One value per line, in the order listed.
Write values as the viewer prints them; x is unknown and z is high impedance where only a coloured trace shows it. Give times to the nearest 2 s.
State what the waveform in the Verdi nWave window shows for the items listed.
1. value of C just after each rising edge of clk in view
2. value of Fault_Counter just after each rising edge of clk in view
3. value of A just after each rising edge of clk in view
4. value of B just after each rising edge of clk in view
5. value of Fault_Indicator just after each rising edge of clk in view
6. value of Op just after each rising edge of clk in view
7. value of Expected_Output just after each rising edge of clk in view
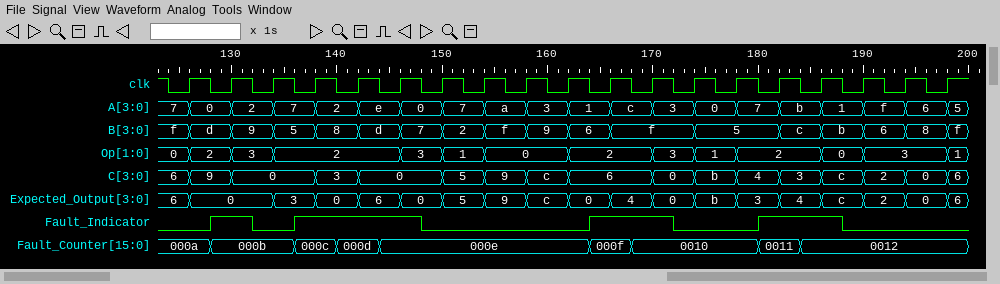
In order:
9, 0, 0, 3, 0, 0, 5, 9, c, 6, 6, 0, b, 4, 3, c, 2, 0, 6
000a, 000b, 000b, 000c, 000d, 000e, 000e, 000e, 000e, 000e, 000f, 0010, 0010, 0010, 0011, 0012, 0012, 0012, 0012
0, 2, 7, 2, e, 0, 7, a, 3, 1, c, 3, 0, 7, b, 1, f, 6, 5
d, 9, 5, 8, d, 7, 2, f, 9, 6, f, f, 5, 5, c, b, 6, 8, f
0 1 0 1 1 1 0 0 0 0 1 1 0 0 1 1 0 0 0
2, 3, 2, 2, 2, 3, 1, 0, 0, 2, 2, 3, 1, 2, 2, 0, 3, 3, 1
0, 0, 3, 0, 6, 0, 5, 9, c, 0, 4, 0, b, 3, 4, c, 2, 0, 6
